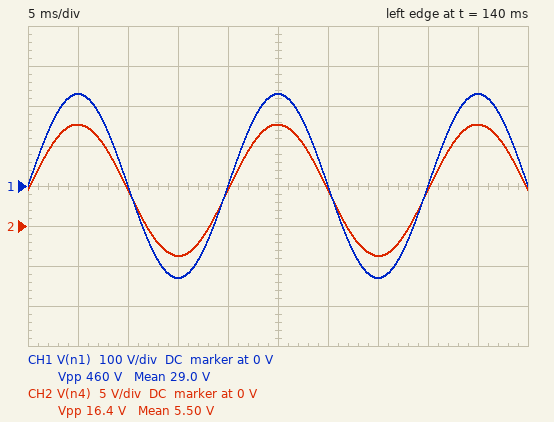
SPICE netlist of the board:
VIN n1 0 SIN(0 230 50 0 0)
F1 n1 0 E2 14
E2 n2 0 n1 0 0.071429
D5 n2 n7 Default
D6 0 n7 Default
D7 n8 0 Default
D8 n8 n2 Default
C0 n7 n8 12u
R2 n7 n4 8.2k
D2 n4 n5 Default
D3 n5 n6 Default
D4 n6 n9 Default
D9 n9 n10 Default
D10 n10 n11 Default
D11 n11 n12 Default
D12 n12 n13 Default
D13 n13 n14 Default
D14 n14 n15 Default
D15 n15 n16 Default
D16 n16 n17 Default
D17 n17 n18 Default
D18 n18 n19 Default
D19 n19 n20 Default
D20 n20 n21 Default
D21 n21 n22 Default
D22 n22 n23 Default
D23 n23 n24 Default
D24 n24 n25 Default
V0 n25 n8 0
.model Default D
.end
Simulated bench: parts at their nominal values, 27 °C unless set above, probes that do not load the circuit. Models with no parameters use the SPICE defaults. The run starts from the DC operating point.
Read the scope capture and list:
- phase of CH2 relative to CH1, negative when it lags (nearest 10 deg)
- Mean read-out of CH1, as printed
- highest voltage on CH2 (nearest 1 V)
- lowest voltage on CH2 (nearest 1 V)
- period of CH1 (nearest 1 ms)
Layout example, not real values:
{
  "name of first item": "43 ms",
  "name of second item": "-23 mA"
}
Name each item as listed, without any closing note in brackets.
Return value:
{
  "phase of CH2 relative to CH1, negative when it lags": "0 deg",
  "Mean read-out of CH1, as printed": "29.0 V",
  "highest voltage on CH2": "13 V",
  "lowest voltage on CH2": "-4 V",
  "period of CH1": "20 ms"
}
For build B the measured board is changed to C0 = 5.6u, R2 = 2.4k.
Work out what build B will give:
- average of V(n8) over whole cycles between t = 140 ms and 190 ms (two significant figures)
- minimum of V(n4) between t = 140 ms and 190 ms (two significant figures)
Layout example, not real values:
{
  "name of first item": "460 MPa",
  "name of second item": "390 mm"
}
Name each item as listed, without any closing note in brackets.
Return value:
{
  "average of V(n8) over whole cycles between t = 140 ms and 190 ms": "-7.2 V",
  "minimum of V(n4) between t = 140 ms and 190 ms": "-3.3 V"
}
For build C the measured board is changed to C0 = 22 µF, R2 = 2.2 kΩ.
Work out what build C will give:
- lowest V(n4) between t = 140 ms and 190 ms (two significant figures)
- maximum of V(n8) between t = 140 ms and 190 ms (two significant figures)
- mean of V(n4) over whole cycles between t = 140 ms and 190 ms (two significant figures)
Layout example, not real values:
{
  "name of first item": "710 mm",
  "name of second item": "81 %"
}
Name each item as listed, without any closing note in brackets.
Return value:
{
  "lowest V(n4) between t = 140 ms and 190 ms": "-3.2 V",
  "maximum of V(n8) between t = 140 ms and 190 ms": "730 mV",
  "mean of V(n4) over whole cycles between t = 140 ms and 190 ms": "5.1 V"
}
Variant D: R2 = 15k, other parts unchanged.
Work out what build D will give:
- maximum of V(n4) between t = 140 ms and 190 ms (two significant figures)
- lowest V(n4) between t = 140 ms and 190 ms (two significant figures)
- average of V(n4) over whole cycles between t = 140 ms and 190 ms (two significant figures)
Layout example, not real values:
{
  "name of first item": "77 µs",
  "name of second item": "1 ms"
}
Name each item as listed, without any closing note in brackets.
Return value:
{
  "maximum of V(n4) between t = 140 ms and 190 ms": "12 V",
  "lowest V(n4) between t = 140 ms and 190 ms": "-4.0 V",
  "average of V(n4) over whole cycles between t = 140 ms and 190 ms": "4.2 V"
}
